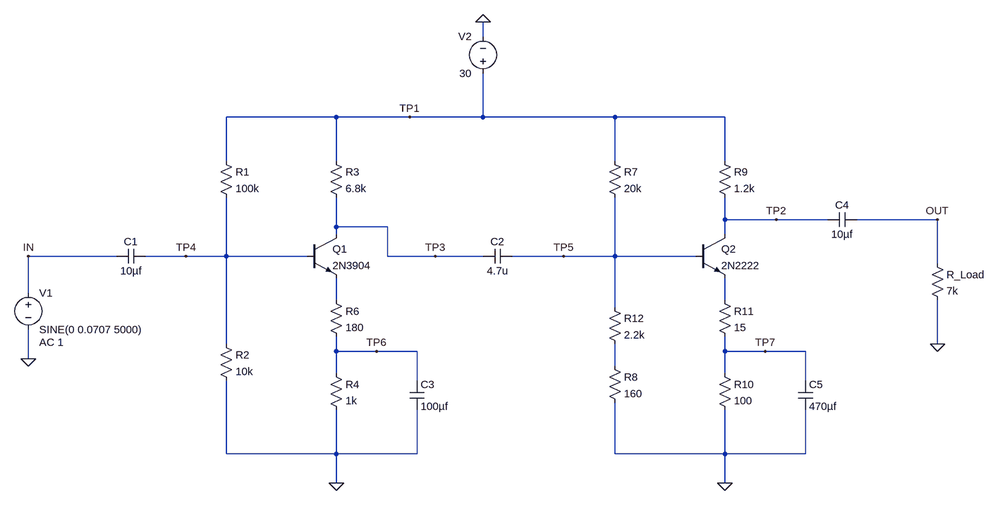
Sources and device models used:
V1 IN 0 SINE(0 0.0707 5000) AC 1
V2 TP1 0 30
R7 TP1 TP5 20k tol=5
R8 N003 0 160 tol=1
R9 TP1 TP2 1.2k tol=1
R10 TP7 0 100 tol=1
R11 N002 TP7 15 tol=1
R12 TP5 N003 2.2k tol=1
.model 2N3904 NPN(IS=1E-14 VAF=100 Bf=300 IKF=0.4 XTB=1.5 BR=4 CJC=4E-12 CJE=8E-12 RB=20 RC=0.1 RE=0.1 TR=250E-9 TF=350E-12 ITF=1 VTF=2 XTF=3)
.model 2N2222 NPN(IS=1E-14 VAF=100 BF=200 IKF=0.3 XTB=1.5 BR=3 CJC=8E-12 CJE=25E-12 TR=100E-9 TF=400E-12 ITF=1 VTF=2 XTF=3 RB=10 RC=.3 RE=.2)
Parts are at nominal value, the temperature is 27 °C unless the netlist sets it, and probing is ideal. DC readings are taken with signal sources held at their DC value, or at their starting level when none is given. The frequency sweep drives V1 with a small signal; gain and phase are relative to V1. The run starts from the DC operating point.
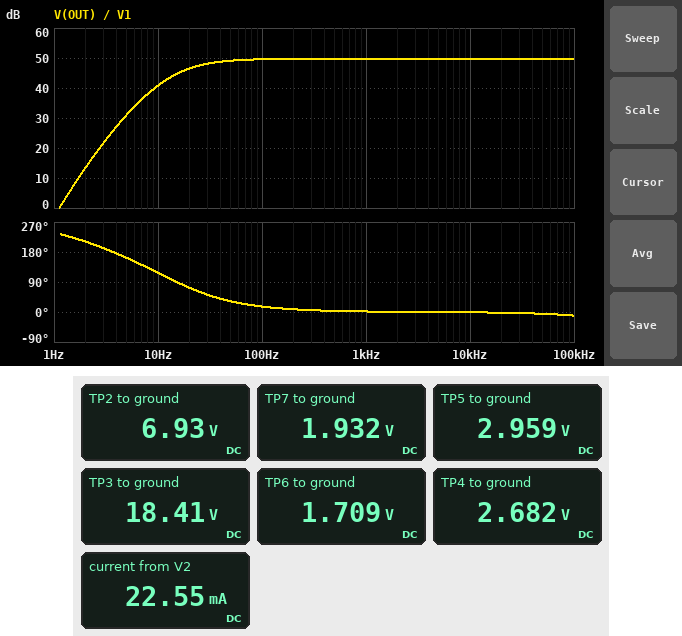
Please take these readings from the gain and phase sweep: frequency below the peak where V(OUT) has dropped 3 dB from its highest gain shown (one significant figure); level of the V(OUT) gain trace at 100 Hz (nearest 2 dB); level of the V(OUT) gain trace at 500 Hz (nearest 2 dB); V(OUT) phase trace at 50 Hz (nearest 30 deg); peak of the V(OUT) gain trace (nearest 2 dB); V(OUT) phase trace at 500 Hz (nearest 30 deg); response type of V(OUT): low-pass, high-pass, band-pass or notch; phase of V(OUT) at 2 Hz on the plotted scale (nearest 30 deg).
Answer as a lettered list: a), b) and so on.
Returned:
a) 20 Hz
b) 50 dB
c) 50 dB
d) 30 deg
e) 50 dB
f) 0 deg
g) high-pass
h) 210 deg
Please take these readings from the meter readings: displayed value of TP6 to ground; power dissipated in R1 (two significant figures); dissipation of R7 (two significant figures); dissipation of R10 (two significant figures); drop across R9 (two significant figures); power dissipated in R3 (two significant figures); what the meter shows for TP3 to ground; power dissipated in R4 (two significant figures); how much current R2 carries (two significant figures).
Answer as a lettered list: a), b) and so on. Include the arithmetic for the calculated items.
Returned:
a) 1.709 V
b) (30 V - 2.682 V)^2 / 100 kΩ = 7.5 mW
c) (30 V - 2.959 V)^2 / 20 kΩ = 37 mW
d) (1.932 V)^2 / 100 Ω = 37 mW
e) 30 V - 6.93 V = 23 V
f) (30 V - 18.41 V)^2 / 6.8 kΩ = 20 mW
g) 18.41 V
h) (1.709 V)^2 / 1 kΩ = 2.9 mW
i) (2.682 V) / 10 kΩ = 270 µA
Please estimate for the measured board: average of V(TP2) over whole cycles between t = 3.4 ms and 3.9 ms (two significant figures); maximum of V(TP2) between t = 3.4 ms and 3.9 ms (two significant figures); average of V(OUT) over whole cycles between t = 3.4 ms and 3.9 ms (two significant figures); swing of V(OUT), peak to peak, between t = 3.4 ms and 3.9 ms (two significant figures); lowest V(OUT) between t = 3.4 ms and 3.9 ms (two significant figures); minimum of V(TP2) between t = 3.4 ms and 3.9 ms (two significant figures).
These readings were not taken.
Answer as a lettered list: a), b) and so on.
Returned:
a) 11 V
b) 26 V
c) 3.9 V
d) 24 V
e) -4.8 V
f) 2.4 V
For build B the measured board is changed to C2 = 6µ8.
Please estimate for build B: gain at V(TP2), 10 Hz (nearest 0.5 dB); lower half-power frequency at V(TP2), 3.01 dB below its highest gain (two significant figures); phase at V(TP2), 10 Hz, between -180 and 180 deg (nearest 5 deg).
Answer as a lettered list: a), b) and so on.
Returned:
a) 41.5 dB
b) 20 Hz
c) 100 deg
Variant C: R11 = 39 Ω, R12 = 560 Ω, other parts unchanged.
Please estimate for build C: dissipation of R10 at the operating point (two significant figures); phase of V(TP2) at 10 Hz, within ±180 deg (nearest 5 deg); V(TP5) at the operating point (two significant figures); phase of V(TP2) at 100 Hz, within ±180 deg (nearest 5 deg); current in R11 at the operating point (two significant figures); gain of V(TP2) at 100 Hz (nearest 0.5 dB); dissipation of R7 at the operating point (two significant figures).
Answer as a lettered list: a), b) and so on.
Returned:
a) 670 µW
b) 95 deg
c) 1.0 V
d) 10 deg
e) 2.6 mA
f) 36.0 dB
g) 42 mW
